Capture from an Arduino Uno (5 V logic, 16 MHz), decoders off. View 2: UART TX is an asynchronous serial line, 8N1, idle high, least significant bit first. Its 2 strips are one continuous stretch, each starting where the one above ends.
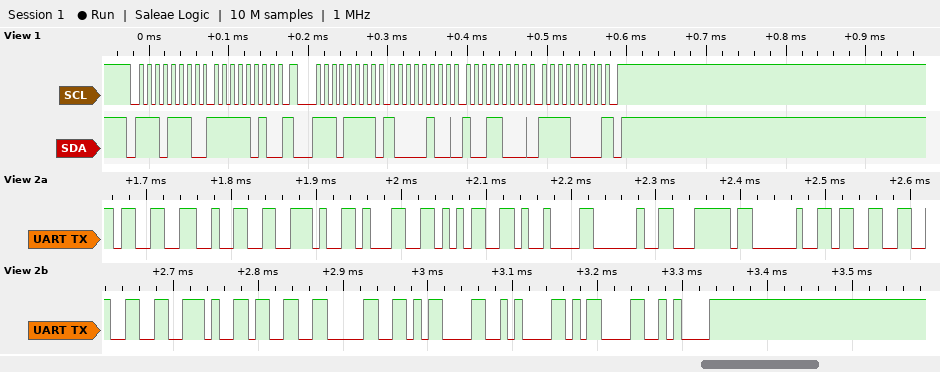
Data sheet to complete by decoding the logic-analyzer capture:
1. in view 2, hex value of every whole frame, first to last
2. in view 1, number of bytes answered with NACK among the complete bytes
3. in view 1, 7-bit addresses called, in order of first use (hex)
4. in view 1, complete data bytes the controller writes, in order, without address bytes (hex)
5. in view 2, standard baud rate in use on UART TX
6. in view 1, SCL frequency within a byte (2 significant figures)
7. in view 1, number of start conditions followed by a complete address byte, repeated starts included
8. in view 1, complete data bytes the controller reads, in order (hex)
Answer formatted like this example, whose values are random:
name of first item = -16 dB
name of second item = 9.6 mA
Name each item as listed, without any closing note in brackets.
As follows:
in view 2, hex value of every whole frame, first to last = 33 32 2E 31 35 09 20 7C 20 33 32 2E 33 30 0D 0A 0D 0A
in view 1, number of bytes answered with NACK among the complete bytes = 1
in view 1, 7-bit addresses called, in order of first use = 0x77
in view 1, complete data bytes the controller writes, in order, without address bytes = FA
in view 2, standard baud rate in use on UART TX = 115200 baud
in view 1, SCL frequency within a byte = 100 kHz
in view 1, number of start conditions followed by a complete address byte, repeated starts included = 2
in view 1, complete data bytes the controller reads, in order = 84 98 F0
